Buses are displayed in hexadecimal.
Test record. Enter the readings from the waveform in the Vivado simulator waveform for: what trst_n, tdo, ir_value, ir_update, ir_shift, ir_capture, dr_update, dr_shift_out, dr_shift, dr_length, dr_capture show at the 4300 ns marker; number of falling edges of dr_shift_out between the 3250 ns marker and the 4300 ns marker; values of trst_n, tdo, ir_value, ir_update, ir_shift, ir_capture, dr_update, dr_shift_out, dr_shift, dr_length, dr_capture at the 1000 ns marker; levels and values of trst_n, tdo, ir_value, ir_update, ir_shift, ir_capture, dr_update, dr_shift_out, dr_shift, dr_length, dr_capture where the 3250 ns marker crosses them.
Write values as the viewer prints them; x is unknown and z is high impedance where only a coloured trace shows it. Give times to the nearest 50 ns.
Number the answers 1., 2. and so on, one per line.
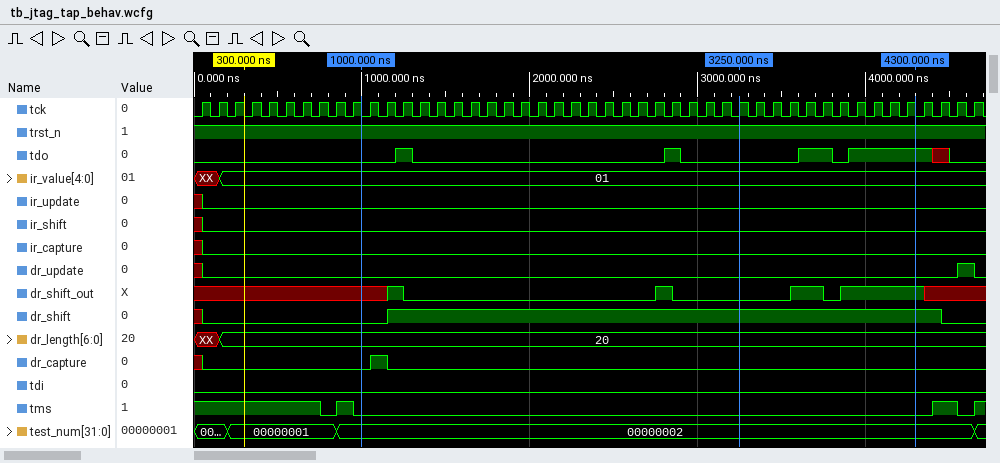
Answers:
1. trst_n=1, tdo=1, ir_value=01, ir_update=0, ir_shift=0, ir_capture=0, dr_update=0, dr_shift_out=1, dr_shift=1, dr_length=20, dr_capture=0
2. 1
3. trst_n=1, tdo=0, ir_value=01, ir_update=0, ir_shift=0, ir_capture=0, dr_update=0, dr_shift_out=x, dr_shift=0, dr_length=20, dr_capture=0
4. trst_n=1, tdo=0, ir_value=01, ir_update=0, ir_shift=0, ir_capture=0, dr_update=0, dr_shift_out=0, dr_shift=1, dr_length=20, dr_capture=0
